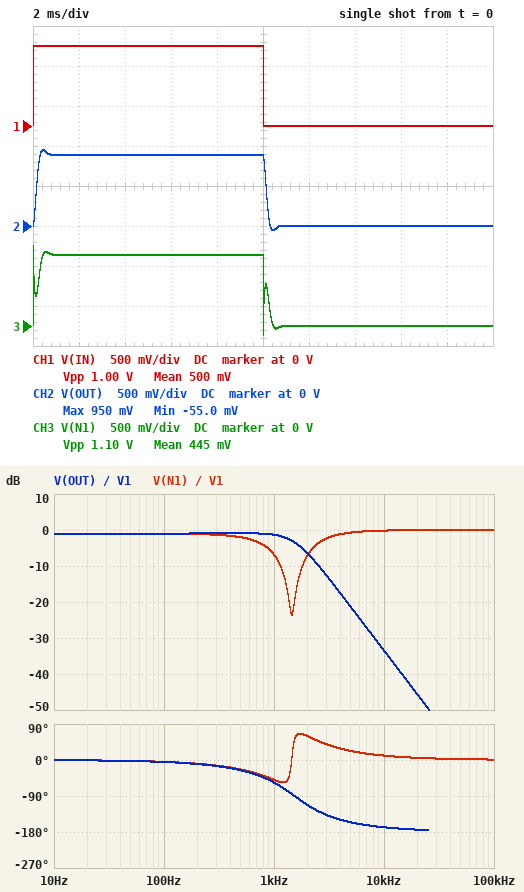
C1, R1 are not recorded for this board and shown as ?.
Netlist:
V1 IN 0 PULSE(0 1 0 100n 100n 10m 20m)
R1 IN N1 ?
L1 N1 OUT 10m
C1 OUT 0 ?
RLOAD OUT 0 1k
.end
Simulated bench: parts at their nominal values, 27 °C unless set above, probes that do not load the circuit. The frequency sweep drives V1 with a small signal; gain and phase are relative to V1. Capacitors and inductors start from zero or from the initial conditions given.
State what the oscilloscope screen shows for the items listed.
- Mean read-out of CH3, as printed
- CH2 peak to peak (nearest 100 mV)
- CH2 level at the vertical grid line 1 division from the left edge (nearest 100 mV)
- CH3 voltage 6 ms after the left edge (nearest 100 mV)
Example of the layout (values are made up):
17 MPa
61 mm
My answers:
445 mV
1.0 V
900 mV
900 mV
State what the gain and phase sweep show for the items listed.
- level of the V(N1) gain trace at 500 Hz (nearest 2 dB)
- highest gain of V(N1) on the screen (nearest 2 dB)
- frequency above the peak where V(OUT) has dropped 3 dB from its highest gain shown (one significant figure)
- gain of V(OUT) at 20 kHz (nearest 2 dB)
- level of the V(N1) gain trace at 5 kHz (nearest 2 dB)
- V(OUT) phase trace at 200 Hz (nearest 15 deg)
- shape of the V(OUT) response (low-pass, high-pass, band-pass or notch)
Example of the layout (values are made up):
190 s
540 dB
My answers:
-2 dB
0 dB
2 kHz
-46 dB
0 dB
-15 deg
low-pass
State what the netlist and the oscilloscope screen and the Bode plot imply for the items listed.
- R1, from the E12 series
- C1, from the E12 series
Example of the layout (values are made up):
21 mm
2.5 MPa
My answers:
120 Ω
1.2 µF
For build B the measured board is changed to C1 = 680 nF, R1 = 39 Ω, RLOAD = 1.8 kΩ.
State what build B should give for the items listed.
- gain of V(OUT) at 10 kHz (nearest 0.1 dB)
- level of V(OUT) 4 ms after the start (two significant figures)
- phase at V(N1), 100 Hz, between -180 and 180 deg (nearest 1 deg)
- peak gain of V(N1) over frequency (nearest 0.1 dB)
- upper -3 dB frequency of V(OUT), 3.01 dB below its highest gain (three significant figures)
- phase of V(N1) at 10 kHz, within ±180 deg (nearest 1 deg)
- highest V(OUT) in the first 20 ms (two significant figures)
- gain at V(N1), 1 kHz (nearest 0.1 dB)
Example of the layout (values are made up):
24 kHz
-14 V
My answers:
-28.3 dB
980 mV
-1 deg
0 dB
2.23 kHz
4 deg
1.5 V
-0.5 dB
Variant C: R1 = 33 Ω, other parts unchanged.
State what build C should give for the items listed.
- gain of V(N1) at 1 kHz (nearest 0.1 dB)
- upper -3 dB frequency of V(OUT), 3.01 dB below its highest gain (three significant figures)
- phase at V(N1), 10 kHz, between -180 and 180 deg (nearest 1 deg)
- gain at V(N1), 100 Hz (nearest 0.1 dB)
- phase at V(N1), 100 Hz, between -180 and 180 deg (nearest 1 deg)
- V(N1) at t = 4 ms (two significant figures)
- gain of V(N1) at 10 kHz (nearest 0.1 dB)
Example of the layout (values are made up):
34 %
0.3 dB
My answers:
-1.6 dB
1.71 kHz
3 deg
-0.3 dB
-1 deg
970 mV
0 dB
